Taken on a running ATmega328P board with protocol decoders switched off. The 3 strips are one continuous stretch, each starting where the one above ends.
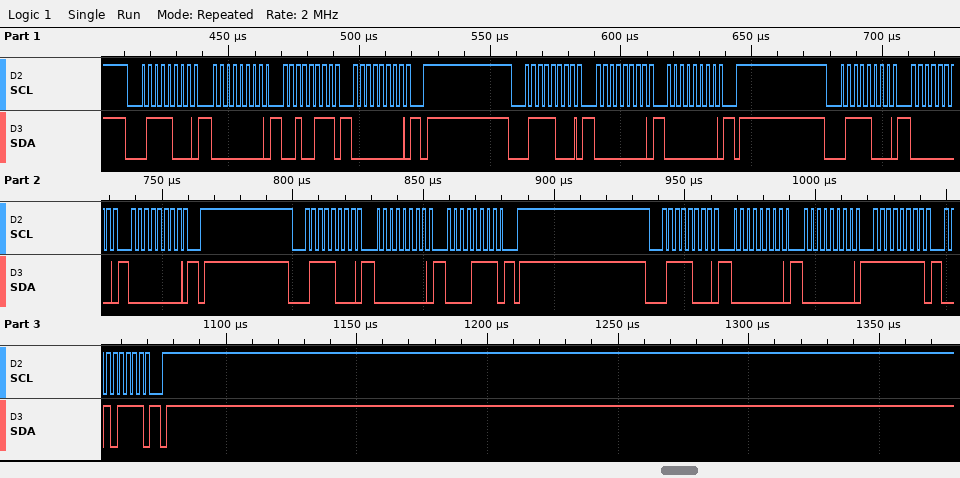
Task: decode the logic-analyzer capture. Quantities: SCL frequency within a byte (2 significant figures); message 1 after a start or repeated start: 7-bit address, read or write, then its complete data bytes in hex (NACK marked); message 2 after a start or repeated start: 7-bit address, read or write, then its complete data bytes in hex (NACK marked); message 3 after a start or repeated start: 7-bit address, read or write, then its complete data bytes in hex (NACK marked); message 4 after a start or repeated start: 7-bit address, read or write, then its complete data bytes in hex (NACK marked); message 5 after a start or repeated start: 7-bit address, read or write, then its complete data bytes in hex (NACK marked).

400 kHz
0x3C write: 00 27 00
0x3C write: 00 00
0x3C write: 00 00
0x3C write: 00 0F
0x3C write: 00 00 FF 2F
